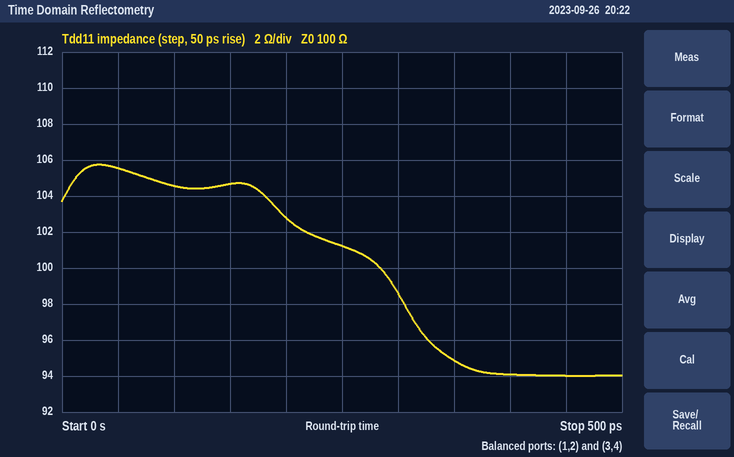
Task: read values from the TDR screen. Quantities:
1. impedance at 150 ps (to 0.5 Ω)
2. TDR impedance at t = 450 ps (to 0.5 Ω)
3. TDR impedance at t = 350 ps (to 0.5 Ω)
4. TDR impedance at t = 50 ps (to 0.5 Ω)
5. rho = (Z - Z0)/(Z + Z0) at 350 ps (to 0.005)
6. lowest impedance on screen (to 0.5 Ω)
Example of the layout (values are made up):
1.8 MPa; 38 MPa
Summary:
104.5 Ω; 94.0 Ω; 95.0 Ω; 105.5 Ω; -0.025; 94.0 Ω
